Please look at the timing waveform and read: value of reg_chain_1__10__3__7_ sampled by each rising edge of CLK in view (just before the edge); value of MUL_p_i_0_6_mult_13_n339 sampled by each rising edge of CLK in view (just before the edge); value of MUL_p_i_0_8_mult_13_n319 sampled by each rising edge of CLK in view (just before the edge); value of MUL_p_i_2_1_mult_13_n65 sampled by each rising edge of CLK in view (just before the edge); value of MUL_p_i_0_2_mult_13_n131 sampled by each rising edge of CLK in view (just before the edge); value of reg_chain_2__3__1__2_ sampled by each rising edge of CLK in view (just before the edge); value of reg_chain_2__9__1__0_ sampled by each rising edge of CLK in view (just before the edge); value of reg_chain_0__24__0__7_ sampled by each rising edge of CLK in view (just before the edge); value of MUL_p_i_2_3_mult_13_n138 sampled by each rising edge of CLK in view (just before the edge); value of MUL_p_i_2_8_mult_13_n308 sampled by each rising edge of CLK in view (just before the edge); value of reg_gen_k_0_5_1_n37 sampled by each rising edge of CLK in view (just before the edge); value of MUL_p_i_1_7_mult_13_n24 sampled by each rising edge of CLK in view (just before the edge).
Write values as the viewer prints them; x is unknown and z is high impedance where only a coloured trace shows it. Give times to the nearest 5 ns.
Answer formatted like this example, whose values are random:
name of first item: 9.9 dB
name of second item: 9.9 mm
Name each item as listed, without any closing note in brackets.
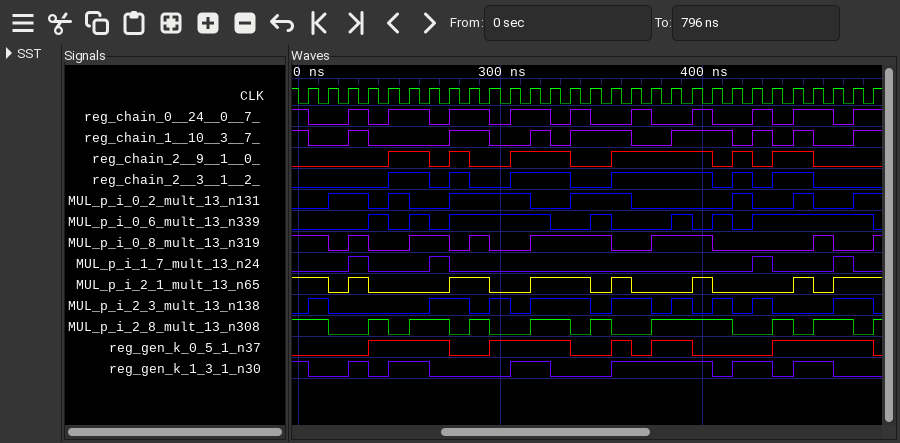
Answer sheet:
value of reg_chain_1__10__3__7_ sampled by each rising edge of CLK in view: 1 0 0 1 0 0 0 0 1 1 0 0 1 0 1 1 1 0 0 1 1 1 0 1 0 1 0 0 1
value of MUL_p_i_0_6_mult_13_n339 sampled by each rising edge of CLK in view: 0 0 0 0 1 0 1 0 1 1 1 1 1 0 0 1 0 0 0 1 0 1 0 1 1 1 1 1 1
value of MUL_p_i_0_8_mult_13_n319 sampled by each rising edge of CLK in view: 1 1 0 1 0 0 1 1 0 1 0 0 1 1 1 1 0 0 1 1 1 0 0 0 0 0 1 0 0
value of MUL_p_i_2_1_mult_13_n65 sampled by each rising edge of CLK in view: 1 1 0 1 0 0 0 0 1 1 0 0 1 1 1 0 1 0 0 0 1 0 0 0 0 1 0 1 1
value of MUL_p_i_0_2_mult_13_n131 sampled by each rising edge of CLK in view: 0 0 1 1 0 1 0 0 1 1 1 1 0 0 1 1 1 0 0 0 0 0 1 0 0 1 0 0 1
value of reg_chain_2__3__1__2_ sampled by each rising edge of CLK in view: 0 0 0 0 0 1 1 0 1 0 0 1 1 1 0 0 1 1 1 1 1 0 1 0 1 1 0 0 0
value of reg_chain_2__9__1__0_ sampled by each rising edge of CLK in view: 0 0 0 0 0 1 1 0 1 0 0 1 1 1 0 0 1 1 1 1 1 0 1 0 1 1 0 0 0
value of reg_chain_0__24__0__7_ sampled by each rising edge of CLK in view: 1 0 0 1 0 1 1 0 1 1 0 1 1 0 1 0 0 1 0 0 1 0 0 1 0 1 1 0 1
value of MUL_p_i_2_3_mult_13_n138 sampled by each rising edge of CLK in view: 0 1 0 0 0 0 0 1 1 0 1 0 1 1 1 0 1 1 0 1 0 1 0 1 0 0 0 1 1
value of MUL_p_i_2_8_mult_13_n308 sampled by each rising edge of CLK in view: 1 1 0 0 1 0 1 1 0 1 0 0 1 1 0 1 0 0 1 1 1 1 0 0 1 0 1 1 0
value of reg_gen_k_0_5_1_n37 sampled by each rising edge of CLK in view: 0 0 0 0 1 1 1 1 0 0 1 1 1 1 0 0 1 0 1 1 0 0 0 0 1 1 1 1 1
value of MUL_p_i_1_7_mult_13_n24 sampled by each rising edge of CLK in view: 0 0 0 1 0 0 0 1 0 0 0 0 0 0 0 0 0 0 0 0 0 0 0 1 0 0 0 1 0
